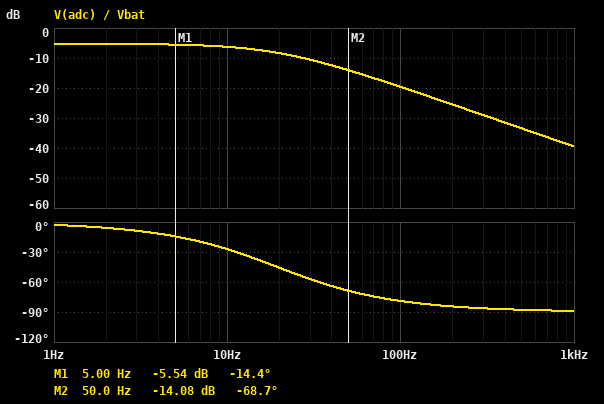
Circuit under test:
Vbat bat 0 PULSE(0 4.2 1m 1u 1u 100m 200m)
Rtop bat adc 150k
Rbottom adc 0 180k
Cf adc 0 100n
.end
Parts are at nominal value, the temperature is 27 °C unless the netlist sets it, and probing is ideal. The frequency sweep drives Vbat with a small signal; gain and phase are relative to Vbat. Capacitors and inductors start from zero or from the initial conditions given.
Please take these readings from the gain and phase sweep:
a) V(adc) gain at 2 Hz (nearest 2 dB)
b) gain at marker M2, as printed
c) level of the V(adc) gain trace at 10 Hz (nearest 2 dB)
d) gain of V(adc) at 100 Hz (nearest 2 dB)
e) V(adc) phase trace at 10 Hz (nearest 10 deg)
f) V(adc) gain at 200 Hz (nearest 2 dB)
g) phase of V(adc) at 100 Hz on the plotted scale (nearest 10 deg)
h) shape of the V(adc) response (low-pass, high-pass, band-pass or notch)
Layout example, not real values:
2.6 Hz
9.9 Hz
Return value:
-6 dB
-14.08 dB
-6 dB
-20 dB
-30 deg
-26 dB
-80 deg
low-pass
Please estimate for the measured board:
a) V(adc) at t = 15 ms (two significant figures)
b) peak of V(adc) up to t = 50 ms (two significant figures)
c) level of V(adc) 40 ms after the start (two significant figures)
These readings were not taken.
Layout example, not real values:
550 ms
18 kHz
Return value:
1.9 V
2.3 V
2.3 V
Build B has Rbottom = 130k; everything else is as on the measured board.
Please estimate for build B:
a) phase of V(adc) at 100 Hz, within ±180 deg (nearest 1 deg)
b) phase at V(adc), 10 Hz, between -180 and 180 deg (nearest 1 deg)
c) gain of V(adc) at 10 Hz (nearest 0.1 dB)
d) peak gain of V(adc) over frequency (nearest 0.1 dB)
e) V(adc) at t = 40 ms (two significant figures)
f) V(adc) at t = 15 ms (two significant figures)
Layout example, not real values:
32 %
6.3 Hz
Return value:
-77 deg
-24 deg
-7.4 dB
-6.7 dB
1.9 V
1.7 V
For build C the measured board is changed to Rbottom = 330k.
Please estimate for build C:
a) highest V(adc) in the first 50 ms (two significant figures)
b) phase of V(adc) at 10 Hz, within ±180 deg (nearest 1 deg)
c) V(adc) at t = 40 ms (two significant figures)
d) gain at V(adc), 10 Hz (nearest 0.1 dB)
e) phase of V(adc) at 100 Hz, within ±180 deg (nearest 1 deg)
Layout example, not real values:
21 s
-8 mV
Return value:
2.9 V
-33 deg
2.8 V
-4.8 dB
-81 deg
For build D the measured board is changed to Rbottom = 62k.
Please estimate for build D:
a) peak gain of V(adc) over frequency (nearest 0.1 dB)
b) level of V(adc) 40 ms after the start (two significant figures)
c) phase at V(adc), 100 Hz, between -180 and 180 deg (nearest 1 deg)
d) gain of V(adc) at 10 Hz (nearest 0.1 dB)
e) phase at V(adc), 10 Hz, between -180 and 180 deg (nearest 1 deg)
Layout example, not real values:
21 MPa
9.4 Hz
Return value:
-10.7 dB
1.2 V
-70 deg
-11.0 dB
-15 deg
